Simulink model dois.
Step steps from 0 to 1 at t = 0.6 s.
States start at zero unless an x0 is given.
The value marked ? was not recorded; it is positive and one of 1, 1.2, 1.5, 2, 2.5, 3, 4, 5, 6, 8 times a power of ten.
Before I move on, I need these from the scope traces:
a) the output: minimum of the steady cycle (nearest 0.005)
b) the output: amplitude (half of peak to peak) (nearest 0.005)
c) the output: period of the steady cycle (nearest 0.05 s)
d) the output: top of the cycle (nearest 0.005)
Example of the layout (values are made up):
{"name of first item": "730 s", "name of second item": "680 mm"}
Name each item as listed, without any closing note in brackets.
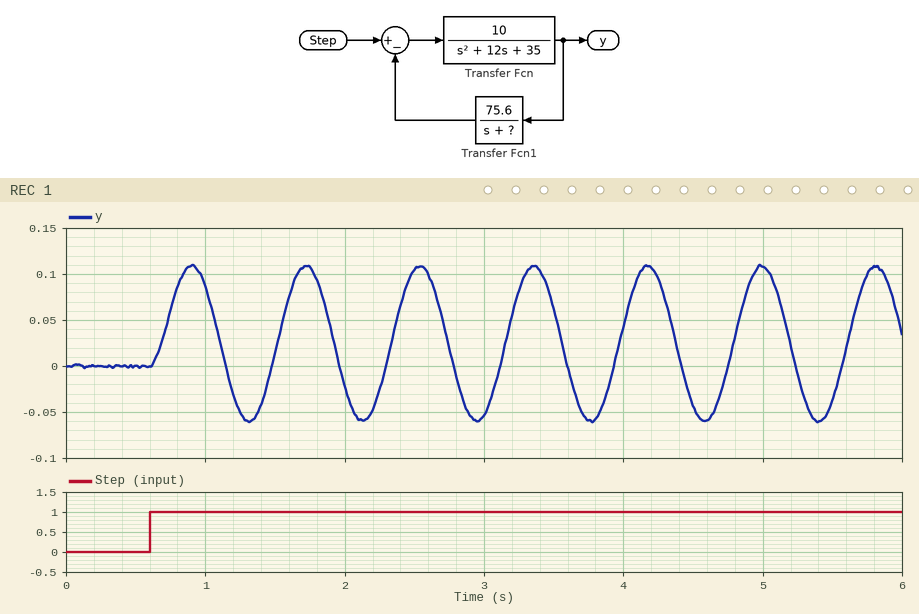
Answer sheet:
{"the output: minimum of the steady cycle": "-0.060", "the output: amplitude (half of peak to peak)": "0.085", "the output: period of the steady cycle": "0.80 s", "the output: top of the cycle": "0.110"}
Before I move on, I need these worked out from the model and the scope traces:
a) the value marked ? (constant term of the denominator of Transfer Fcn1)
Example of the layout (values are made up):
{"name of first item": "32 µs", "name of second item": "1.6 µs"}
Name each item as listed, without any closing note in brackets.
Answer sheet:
{"the value marked ?": "2"}
